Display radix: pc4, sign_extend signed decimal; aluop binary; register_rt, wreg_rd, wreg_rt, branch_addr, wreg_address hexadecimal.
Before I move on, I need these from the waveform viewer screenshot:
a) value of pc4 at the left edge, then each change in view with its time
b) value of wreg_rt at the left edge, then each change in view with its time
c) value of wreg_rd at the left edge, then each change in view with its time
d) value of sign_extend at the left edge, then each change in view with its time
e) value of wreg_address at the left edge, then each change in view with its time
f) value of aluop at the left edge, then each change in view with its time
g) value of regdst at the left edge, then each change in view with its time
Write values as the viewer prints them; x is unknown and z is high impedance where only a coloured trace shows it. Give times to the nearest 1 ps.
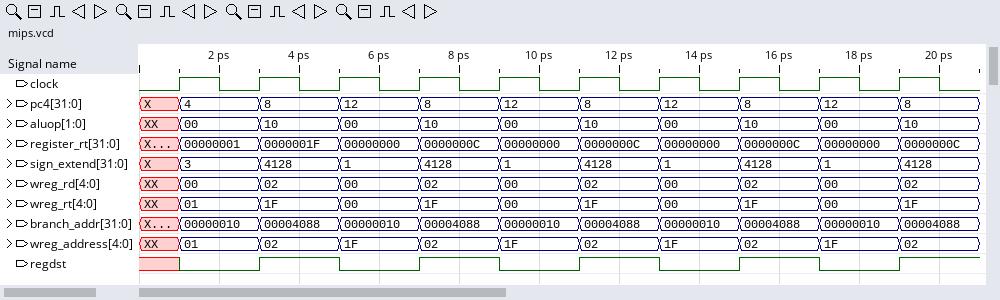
X, 4 at 1 ps, 8 at 3 ps, 12 at 5 ps, 8 at 7 ps, 12 at 9 ps, 8 at 11 ps, 12 at 13 ps, 8 at 15 ps, 12 at 17 ps, 8 at 19 ps
XX, 01 at 1 ps, 1F at 3 ps, 00 at 5 ps, 1F at 7 ps, 00 at 9 ps, 1F at 11 ps, 00 at 13 ps, 1F at 15 ps, 00 at 17 ps, 1F at 19 ps
XX, 00 at 1 ps, 02 at 3 ps, 00 at 5 ps, 02 at 7 ps, 00 at 9 ps, 02 at 11 ps, 00 at 13 ps, 02 at 15 ps, 00 at 17 ps, 02 at 19 ps
X, 3 at 1 ps, 4128 at 3 ps, 1 at 5 ps, 4128 at 7 ps, 1 at 9 ps, 4128 at 11 ps, 1 at 13 ps, 4128 at 15 ps, 1 at 17 ps, 4128 at 19 ps
XX, 01 at 1 ps, 02 at 3 ps, 1F at 5 ps, 02 at 7 ps, 1F at 9 ps, 02 at 11 ps, 1F at 13 ps, 02 at 15 ps, 1F at 17 ps, 02 at 19 ps
XX, 00 at 1 ps, 10 at 3 ps, 00 at 5 ps, 10 at 7 ps, 00 at 9 ps, 10 at 11 ps, 00 at 13 ps, 10 at 15 ps, 00 at 17 ps, 10 at 19 ps
x, 0 at 1 ps, 1 at 3 ps, 0 at 5 ps, 1 at 7 ps, 0 at 9 ps, 1 at 11 ps, 0 at 13 ps, 1 at 15 ps, 0 at 17 ps, 1 at 19 ps
